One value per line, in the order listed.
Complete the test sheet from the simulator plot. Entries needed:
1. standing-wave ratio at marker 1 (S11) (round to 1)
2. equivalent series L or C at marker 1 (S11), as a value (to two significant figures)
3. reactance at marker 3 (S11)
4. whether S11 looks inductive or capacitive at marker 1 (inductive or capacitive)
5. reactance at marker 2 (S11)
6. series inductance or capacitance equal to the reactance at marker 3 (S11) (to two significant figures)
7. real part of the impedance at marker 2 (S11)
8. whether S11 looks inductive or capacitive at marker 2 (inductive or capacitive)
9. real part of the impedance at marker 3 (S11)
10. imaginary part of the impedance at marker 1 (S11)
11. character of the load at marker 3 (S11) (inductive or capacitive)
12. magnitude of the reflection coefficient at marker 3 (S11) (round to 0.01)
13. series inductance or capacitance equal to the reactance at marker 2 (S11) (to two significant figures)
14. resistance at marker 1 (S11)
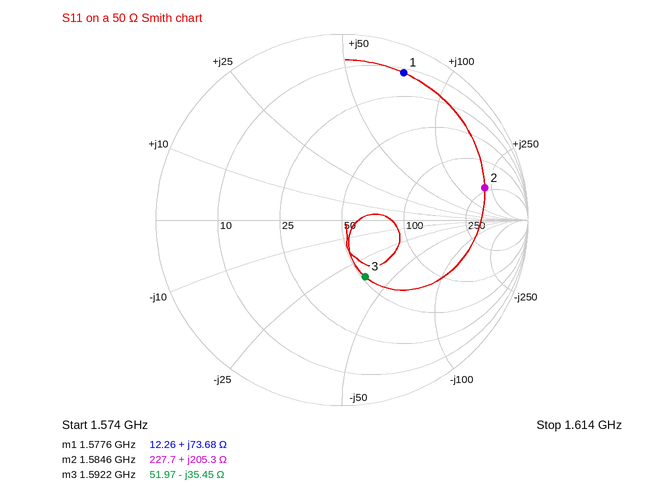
13
7.4 nH
-35.45 Ω
inductive
+205.3 Ω
2.8 pF
227.7 Ω
inductive
51.97 Ω
+73.68 Ω
capacitive
0.33
21 nH
12.26 Ω
